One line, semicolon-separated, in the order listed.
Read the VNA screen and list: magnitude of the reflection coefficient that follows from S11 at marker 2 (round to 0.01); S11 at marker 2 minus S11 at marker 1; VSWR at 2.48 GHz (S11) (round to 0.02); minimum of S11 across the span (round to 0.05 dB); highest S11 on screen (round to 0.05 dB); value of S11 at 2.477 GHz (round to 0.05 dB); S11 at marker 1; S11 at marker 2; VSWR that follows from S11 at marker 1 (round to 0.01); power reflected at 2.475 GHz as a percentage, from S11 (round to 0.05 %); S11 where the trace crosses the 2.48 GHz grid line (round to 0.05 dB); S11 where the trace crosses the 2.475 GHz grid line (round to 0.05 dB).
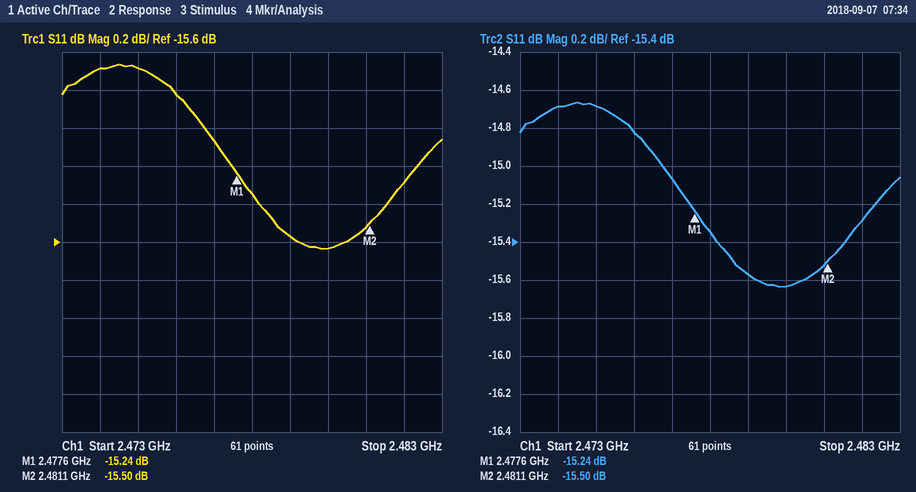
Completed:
0.17; -0.26 dB; 1.40; -15.65 dB; -14.65 dB; -15.05 dB; -15.24 dB; -15.50 dB; 1.42; 3.40 %; -15.65 dB; -14.70 dB
